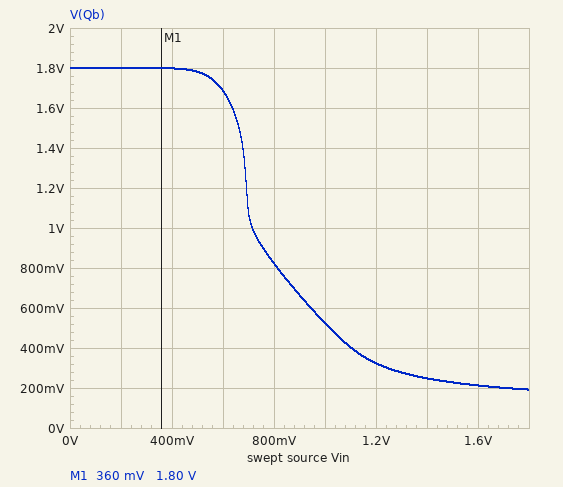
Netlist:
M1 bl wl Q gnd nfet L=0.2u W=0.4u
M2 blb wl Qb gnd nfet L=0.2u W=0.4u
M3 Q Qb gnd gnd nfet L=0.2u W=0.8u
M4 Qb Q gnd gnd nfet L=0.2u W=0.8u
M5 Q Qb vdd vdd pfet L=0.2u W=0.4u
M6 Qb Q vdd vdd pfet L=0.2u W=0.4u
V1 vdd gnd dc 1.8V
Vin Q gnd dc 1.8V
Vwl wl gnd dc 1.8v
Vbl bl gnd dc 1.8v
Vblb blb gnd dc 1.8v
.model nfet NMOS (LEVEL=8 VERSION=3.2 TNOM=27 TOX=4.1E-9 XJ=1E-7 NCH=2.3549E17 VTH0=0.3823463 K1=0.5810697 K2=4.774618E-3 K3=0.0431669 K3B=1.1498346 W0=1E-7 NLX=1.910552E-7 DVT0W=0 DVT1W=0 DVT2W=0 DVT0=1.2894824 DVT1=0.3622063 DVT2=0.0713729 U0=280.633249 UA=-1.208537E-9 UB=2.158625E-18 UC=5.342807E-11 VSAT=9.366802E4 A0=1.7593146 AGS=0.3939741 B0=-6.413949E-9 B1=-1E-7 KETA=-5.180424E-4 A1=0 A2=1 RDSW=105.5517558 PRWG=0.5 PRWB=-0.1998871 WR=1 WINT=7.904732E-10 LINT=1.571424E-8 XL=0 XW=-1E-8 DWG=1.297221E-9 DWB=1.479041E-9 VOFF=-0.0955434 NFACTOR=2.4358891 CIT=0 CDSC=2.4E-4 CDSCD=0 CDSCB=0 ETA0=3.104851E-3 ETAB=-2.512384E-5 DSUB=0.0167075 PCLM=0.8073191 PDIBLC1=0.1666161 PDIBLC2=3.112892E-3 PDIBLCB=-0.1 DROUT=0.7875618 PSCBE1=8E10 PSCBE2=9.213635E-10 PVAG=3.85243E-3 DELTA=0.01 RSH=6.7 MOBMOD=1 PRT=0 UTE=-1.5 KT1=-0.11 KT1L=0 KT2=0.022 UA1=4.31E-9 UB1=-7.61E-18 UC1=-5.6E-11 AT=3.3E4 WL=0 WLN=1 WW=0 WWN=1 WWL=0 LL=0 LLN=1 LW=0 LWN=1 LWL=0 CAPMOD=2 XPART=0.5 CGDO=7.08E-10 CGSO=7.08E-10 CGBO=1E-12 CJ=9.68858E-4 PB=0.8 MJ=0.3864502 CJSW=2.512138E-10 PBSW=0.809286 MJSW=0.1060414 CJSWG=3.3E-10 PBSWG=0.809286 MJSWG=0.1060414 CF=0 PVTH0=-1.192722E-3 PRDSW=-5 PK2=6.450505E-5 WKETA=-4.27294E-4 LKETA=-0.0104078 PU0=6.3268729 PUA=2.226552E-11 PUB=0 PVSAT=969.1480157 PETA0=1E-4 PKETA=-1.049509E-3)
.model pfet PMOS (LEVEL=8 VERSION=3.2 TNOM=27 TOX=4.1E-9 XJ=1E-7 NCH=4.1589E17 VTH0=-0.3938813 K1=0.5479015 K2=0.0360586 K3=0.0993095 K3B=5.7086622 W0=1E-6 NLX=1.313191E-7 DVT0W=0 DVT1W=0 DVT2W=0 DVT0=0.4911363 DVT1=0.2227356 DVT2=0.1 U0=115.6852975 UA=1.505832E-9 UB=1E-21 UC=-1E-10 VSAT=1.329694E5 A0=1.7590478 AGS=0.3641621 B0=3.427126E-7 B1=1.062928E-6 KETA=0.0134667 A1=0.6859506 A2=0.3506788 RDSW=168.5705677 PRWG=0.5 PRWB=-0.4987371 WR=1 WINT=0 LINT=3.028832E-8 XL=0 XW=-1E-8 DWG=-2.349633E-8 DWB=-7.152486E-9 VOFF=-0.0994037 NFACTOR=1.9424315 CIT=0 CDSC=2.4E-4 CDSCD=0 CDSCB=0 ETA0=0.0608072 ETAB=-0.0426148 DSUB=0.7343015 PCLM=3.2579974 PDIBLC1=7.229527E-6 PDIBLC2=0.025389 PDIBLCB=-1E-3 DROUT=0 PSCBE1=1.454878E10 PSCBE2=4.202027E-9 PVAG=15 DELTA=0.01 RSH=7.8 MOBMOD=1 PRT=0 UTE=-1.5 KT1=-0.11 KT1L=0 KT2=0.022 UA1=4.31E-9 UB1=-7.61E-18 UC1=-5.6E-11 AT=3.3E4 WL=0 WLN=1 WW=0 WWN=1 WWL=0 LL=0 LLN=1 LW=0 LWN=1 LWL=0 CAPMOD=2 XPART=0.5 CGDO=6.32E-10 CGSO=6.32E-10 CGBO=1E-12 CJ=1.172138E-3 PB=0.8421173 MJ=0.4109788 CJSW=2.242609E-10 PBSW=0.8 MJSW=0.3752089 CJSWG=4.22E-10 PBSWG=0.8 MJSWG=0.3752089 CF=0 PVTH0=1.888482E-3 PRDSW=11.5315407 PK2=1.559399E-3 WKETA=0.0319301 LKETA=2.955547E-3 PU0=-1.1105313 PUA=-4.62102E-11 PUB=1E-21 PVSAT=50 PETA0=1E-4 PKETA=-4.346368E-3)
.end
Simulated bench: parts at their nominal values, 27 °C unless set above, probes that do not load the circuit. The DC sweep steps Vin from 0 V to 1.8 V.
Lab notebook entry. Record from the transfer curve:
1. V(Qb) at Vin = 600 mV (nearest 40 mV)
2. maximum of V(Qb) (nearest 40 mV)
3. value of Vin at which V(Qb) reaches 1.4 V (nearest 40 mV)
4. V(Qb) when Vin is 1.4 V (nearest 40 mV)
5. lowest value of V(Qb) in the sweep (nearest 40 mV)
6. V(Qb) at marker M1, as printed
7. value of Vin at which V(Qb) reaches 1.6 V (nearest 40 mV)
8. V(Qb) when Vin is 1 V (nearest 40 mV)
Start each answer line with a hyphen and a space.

- 1.68 V
- 1.80 V
- 680 mV
- 240 mV
- 200 mV
- 1.80 V
- 640 mV
- 520 mV
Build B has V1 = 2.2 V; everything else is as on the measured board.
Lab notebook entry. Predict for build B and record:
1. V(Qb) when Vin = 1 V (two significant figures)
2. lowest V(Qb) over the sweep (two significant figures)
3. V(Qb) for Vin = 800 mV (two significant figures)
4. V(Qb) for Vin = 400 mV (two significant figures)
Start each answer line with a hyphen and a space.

- 630 mV
- 190 mV
- 1.1 V
- 2.2 V
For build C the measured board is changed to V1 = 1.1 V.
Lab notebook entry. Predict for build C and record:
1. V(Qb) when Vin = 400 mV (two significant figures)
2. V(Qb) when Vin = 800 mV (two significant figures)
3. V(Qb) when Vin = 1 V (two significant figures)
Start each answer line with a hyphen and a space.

- 1.1 V
- 720 mV
- 490 mV
